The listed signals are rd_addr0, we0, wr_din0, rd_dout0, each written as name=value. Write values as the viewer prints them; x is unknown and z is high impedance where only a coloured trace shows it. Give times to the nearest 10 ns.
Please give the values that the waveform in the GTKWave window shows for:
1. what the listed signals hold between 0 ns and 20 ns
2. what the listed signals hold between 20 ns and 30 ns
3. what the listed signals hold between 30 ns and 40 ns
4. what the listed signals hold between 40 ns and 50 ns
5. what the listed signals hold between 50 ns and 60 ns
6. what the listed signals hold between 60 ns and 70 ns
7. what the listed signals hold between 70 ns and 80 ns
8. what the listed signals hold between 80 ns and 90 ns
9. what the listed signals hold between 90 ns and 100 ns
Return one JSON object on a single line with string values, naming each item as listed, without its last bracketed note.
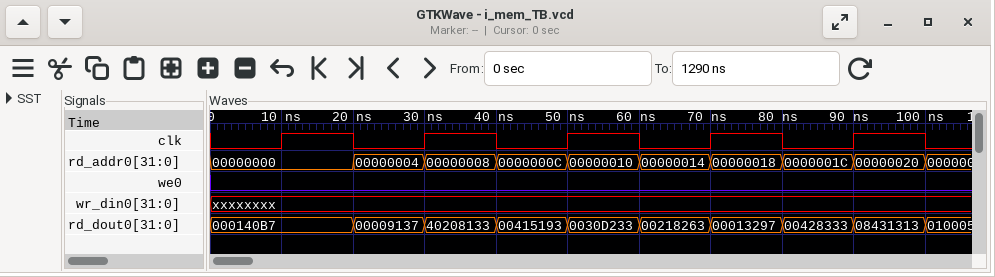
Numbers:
{"what the listed signals hold between 0 ns and 20 ns": "rd_addr0=00000000, we0=0, wr_din0=xxxxxxxx, rd_dout0=000140B7", "what the listed signals hold between 20 ns and 30 ns": "rd_addr0=00000004, we0=0, wr_din0=xxxxxxxx, rd_dout0=00009137", "what the listed signals hold between 30 ns and 40 ns": "rd_addr0=00000008, we0=0, wr_din0=xxxxxxxx, rd_dout0=40208133", "what the listed signals hold between 40 ns and 50 ns": "rd_addr0=0000000C, we0=0, wr_din0=xxxxxxxx, rd_dout0=00415193", "what the listed signals hold between 50 ns and 60 ns": "rd_addr0=00000010, we0=0, wr_din0=xxxxxxxx, rd_dout0=0030D233", "what the listed signals hold between 60 ns and 70 ns": "rd_addr0=00000014, we0=0, wr_din0=xxxxxxxx, rd_dout0=00218263", "what the listed signals hold between 70 ns and 80 ns": "rd_addr0=00000018, we0=0, wr_din0=xxxxxxxx, rd_dout0=00013297", "what the listed signals hold between 80 ns and 90 ns": "rd_addr0=0000001C, we0=0, wr_din0=xxxxxxxx, rd_dout0=00428333", "what the listed signals hold between 90 ns and 100 ns": "rd_addr0=00000020, we0=0, wr_din0=xxxxxxxx, rd_dout0=08431313"}
